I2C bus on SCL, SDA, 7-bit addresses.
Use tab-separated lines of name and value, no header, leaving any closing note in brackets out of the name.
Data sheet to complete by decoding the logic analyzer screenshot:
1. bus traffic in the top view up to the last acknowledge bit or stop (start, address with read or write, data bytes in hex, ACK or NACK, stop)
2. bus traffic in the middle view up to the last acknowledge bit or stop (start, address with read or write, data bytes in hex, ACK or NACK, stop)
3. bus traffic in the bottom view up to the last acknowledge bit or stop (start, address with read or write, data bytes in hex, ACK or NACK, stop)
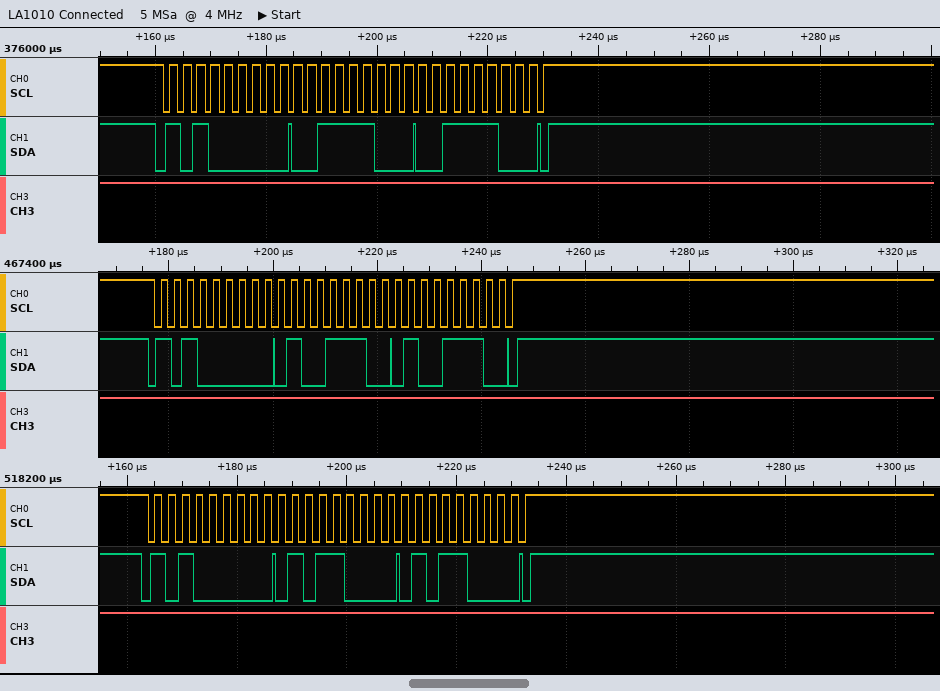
bus traffic in the top view up to the last acknowledge bit or stop	start, address 50 write ACK, 3C ACK, 3C ACK, stop
bus traffic in the middle view up to the last acknowledge bit or stop	start, address 50 write ACK, 4E ACK, 4E ACK, stop
bus traffic in the bottom view up to the last acknowledge bit or stop	start, address 50 write ACK, 58 ACK, 58 ACK, stop
